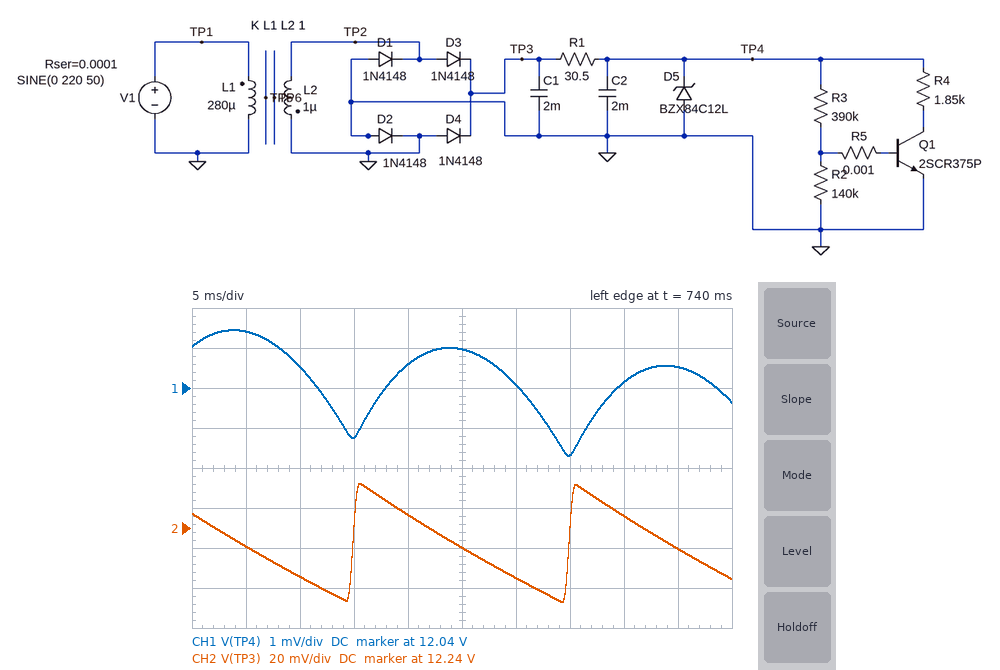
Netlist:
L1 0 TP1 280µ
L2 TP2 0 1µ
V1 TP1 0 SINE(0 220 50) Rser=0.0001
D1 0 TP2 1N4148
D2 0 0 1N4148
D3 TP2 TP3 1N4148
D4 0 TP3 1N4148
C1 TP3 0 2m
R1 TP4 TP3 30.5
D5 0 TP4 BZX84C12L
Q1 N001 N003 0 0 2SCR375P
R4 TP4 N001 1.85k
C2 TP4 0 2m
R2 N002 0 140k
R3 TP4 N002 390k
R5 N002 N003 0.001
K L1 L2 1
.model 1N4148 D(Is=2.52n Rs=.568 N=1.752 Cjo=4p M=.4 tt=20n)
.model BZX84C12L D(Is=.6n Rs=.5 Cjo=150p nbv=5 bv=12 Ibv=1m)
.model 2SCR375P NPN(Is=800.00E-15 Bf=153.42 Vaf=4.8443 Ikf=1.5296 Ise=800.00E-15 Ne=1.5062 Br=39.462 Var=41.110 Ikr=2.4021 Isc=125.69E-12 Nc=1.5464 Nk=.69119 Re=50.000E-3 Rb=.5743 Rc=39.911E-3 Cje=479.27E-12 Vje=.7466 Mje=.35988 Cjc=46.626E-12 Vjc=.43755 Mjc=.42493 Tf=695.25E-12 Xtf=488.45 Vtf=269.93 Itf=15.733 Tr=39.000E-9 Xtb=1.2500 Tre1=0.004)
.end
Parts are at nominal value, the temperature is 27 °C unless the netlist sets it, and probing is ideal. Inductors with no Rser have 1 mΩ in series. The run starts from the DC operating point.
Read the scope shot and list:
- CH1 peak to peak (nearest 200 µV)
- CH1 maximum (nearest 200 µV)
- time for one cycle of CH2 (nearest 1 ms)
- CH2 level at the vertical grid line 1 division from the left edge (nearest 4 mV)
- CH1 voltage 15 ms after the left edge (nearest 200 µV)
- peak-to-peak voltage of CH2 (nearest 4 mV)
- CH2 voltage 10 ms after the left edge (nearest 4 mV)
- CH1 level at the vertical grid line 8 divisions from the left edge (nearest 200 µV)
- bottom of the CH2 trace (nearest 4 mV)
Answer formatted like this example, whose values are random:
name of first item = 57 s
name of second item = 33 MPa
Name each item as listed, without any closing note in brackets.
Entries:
CH1 peak to peak = 3.2 mV
CH1 maximum = 12.0384 V
time for one cycle of CH2 = 20 ms
CH2 level at the vertical grid line 1 division from the left edge = 12.232 V
CH1 voltage 15 ms after the left edge = 12.0358 V
peak-to-peak voltage of CH2 = 60 mV
CH2 voltage 10 ms after the left edge = 12.216 V
CH1 level at the vertical grid line 8 divisions from the left edge = 12.0372 V
bottom of the CH2 trace = 12.204 V
